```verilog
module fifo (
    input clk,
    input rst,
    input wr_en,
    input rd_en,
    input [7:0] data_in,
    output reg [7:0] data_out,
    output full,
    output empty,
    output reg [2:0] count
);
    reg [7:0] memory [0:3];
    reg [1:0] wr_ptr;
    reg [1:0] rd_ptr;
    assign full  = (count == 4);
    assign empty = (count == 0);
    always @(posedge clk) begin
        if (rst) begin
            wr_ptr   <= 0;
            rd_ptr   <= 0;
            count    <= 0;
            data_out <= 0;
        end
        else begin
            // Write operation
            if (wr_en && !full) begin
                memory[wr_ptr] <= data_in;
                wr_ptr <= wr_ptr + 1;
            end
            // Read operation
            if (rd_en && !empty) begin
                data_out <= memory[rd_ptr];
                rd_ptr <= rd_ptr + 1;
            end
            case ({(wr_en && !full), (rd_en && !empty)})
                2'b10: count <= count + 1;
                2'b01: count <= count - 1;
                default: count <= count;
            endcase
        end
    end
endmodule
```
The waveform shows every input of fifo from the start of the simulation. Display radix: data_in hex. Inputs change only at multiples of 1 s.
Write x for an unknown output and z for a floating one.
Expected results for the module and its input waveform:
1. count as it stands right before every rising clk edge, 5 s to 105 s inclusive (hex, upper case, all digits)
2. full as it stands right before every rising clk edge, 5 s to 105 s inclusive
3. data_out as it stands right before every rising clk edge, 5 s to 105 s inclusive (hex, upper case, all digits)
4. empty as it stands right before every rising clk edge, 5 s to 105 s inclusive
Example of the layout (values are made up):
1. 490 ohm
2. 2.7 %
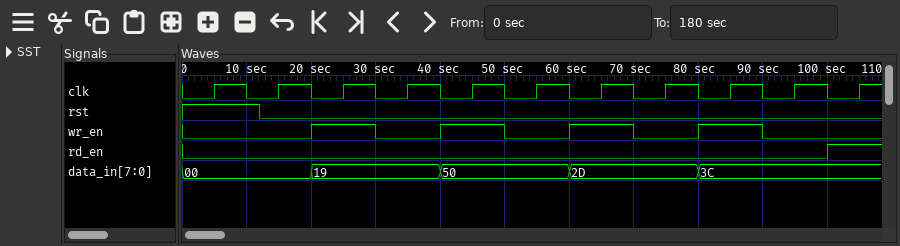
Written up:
1. x, 0, 0, 1, 1, 2, 2, 3, 3, 4, 4
2. x 0 0 0 0 0 0 0 0 1 1
3. x, 00, 00, 00, 00, 00, 00, 00, 00, 00, 00
4. x 1 1 0 0 0 0 0 0 0 0
